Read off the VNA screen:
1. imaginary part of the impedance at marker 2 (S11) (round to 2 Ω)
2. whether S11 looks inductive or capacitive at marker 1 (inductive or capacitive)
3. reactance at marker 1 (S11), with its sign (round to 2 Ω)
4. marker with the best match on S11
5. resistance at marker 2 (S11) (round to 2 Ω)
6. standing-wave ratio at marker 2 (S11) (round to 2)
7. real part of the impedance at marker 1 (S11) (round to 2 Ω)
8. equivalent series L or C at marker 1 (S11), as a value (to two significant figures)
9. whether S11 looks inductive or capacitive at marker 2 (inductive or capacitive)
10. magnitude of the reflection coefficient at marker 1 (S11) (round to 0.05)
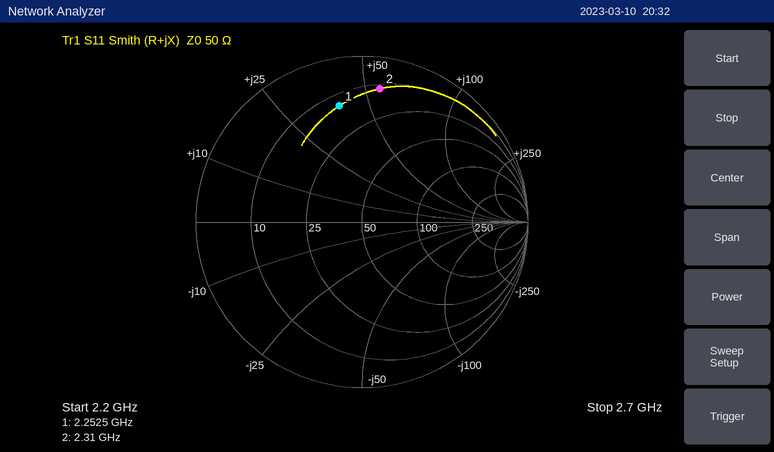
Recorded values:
+56 Ω
inductive
+40 Ω
marker 1
12 Ω
10
14 Ω
2.8 nH
inductive
0.70
